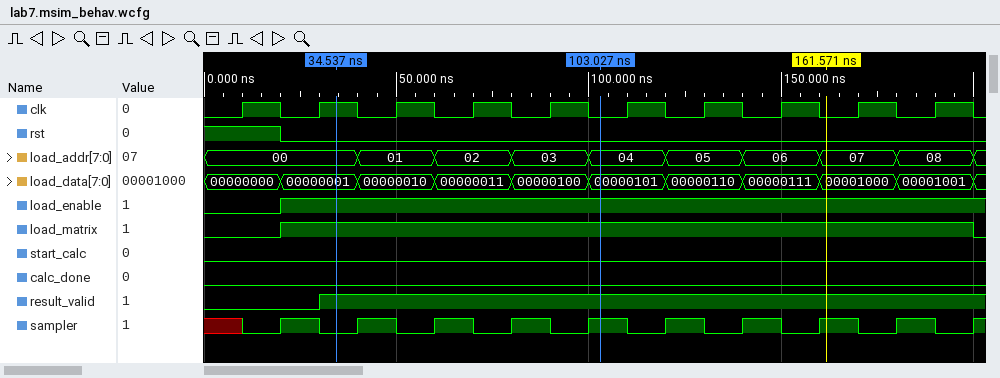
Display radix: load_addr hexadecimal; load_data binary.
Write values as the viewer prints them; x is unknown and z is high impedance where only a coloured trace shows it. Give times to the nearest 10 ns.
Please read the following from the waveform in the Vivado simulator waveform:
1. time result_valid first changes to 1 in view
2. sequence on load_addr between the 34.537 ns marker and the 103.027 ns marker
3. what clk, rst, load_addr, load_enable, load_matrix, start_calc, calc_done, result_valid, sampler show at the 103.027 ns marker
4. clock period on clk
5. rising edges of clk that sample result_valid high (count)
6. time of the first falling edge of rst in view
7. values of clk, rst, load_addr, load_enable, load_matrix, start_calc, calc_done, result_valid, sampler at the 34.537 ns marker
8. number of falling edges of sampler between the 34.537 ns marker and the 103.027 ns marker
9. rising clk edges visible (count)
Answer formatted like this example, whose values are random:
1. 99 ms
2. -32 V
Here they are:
1. 30 ns
2. 00, 01, 02, 03, 04
3. clk=0, rst=0, load_addr=04, load_enable=1, load_matrix=1, start_calc=0, calc_done=0, result_valid=1, sampler=1
4. 20 ns
5. 8
6. 20 ns
7. clk=1, rst=0, load_addr=00, load_enable=1, load_matrix=1, start_calc=0, calc_done=0, result_valid=1, sampler=0
8. 3
9. 10
